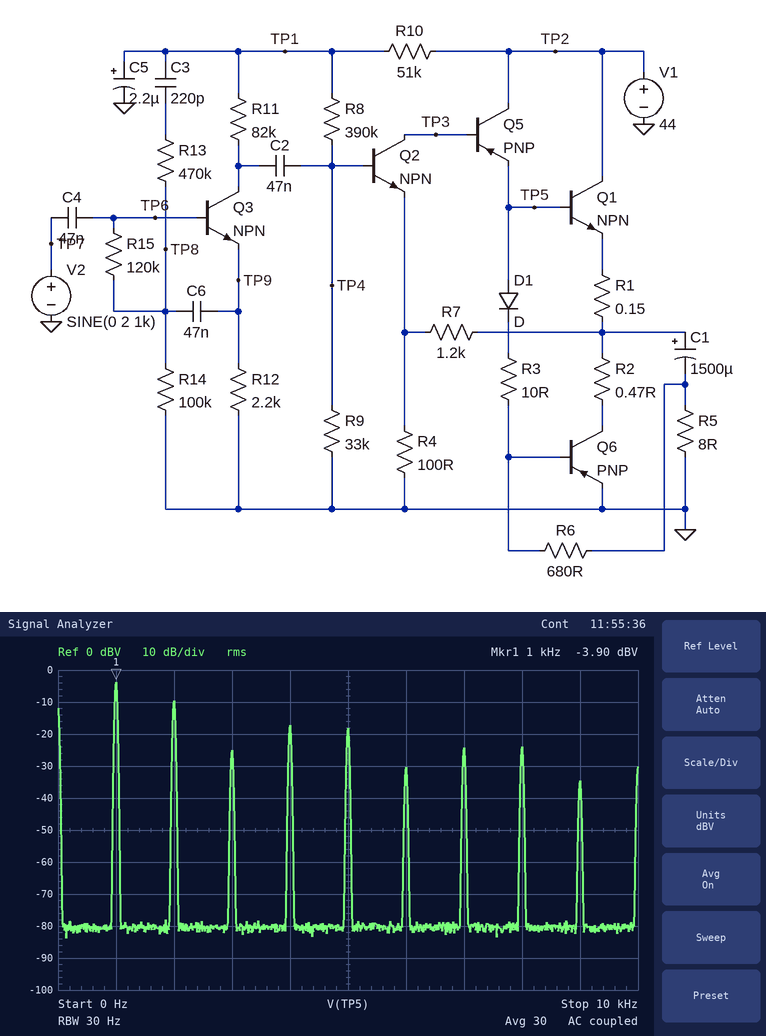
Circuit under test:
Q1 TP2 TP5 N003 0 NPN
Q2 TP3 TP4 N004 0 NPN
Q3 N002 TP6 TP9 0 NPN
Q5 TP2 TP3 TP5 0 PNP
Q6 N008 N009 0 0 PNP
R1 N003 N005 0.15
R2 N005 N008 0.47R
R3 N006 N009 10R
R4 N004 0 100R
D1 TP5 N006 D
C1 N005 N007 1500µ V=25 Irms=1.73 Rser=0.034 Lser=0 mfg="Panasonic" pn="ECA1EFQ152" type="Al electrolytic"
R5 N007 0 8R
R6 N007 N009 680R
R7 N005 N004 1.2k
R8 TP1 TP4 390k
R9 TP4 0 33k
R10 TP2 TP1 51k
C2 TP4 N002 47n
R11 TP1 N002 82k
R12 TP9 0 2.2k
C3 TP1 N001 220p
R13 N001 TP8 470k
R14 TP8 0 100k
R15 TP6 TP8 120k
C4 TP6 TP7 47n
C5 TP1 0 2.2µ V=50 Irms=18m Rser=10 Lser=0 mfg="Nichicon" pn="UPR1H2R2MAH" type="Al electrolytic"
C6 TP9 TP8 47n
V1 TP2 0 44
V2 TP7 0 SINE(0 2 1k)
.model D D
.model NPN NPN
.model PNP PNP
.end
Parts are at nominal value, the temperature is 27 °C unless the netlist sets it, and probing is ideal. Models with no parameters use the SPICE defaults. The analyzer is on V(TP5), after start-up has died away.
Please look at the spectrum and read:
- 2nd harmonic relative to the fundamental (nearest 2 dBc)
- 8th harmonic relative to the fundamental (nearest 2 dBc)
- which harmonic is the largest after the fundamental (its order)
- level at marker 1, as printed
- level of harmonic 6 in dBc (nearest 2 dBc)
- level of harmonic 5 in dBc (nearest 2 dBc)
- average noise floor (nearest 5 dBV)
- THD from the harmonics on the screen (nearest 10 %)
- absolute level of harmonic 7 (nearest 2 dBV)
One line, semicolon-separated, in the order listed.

-6 dBc; -20 dBc; 2; -3.90 dBV; -26 dBc; -14 dBc; -80 dBV; 60 %; -24 dBV
